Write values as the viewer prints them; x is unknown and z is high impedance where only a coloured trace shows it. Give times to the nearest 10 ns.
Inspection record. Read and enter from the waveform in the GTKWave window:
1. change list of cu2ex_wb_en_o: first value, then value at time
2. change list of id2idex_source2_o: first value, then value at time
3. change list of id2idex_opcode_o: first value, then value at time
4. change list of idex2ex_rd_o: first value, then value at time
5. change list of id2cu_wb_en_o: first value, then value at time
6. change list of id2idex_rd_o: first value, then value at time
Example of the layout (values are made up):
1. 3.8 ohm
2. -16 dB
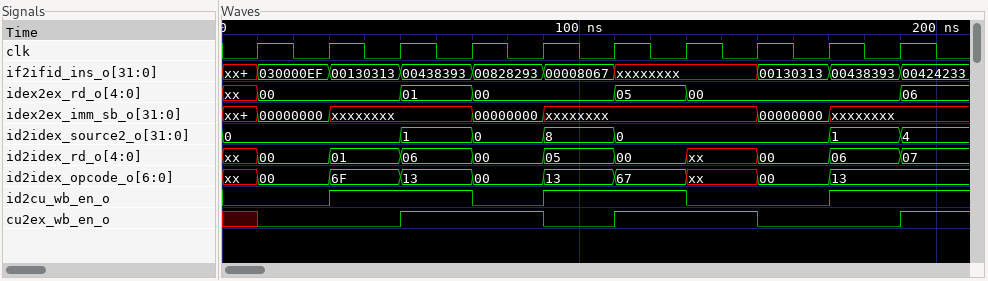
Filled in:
1. x, 0 at 10 ns, 1 at 50 ns, 0 at 90 ns, 1 at 110 ns, 0 at 150 ns, 1 at 190 ns
2. 0, 1 at 50 ns, 0 at 70 ns, 8 at 90 ns, 0 at 110 ns, 1 at 170 ns, 4 at 190 ns
3. xx, 00 at 10 ns, 6F at 30 ns, 13 at 50 ns, 00 at 70 ns, 13 at 90 ns, 67 at 110 ns, xx at 130 ns, 00 at 150 ns, 13 at 170 ns
4. xx, 00 at 10 ns, 01 at 50 ns, 00 at 70 ns, 05 at 110 ns, 00 at 130 ns, 06 at 190 ns
5. 0, 1 at 30 ns, 0 at 70 ns, 1 at 90 ns, 0 at 130 ns, 1 at 170 ns
6. xx, 00 at 10 ns, 01 at 30 ns, 06 at 50 ns, 00 at 70 ns, 05 at 90 ns, 00 at 110 ns, xx at 130 ns, 00 at 150 ns, 06 at 170 ns, 07 at 190 ns
